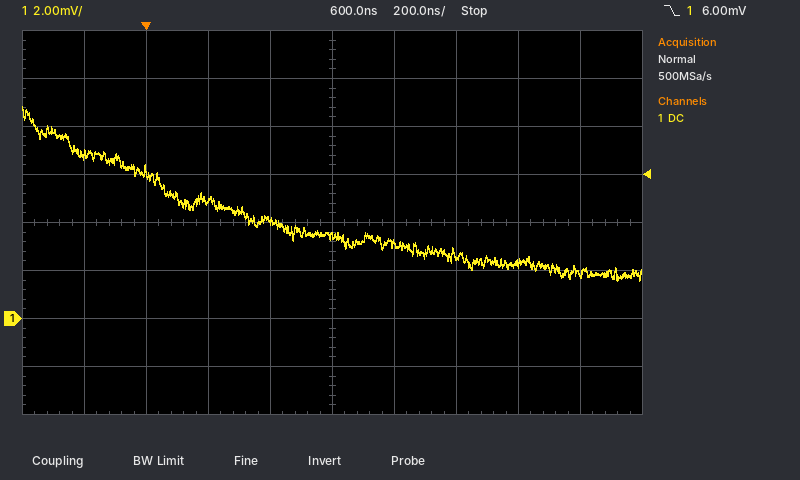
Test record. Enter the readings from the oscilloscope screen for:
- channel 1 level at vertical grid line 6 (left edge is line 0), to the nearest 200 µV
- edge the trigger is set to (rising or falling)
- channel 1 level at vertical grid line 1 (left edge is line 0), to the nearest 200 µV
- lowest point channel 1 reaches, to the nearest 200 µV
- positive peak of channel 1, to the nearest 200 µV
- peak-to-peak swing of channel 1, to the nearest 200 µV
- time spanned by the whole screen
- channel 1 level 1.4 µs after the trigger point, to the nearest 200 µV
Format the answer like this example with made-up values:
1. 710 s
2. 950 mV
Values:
1. 3.2 mV
2. falling
3. 6.8 mV
4. 1.6 mV
5. 8.8 mV
6. 7.2 mV
7. 2 µs
8. 1.8 mV
